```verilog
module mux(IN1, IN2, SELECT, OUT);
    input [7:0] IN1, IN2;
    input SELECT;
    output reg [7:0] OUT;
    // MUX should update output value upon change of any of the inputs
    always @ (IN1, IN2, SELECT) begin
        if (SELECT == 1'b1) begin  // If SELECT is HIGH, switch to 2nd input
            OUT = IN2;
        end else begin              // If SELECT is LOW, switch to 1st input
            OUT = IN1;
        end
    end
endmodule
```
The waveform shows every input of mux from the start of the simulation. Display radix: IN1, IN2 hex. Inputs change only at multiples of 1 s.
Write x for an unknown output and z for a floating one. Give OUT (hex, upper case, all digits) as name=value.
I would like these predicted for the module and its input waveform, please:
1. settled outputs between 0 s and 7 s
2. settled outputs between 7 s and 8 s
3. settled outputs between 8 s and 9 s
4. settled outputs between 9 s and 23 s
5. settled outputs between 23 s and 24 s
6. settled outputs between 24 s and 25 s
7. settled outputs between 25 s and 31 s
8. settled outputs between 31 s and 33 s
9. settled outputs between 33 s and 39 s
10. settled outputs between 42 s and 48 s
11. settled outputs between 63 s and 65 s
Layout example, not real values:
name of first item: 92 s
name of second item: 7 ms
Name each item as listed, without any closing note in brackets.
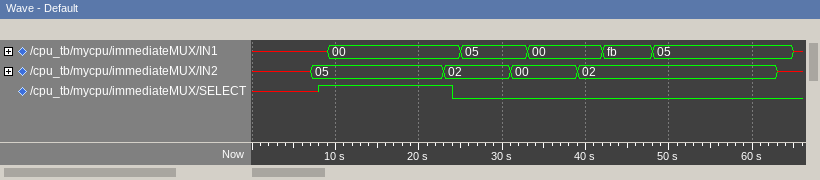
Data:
settled outputs between 0 s and 7 s: OUT=x
settled outputs between 7 s and 8 s: OUT=x
settled outputs between 8 s and 9 s: OUT=05
settled outputs between 9 s and 23 s: OUT=05
settled outputs between 23 s and 24 s: OUT=02
settled outputs between 24 s and 25 s: OUT=00
settled outputs between 25 s and 31 s: OUT=05
settled outputs between 31 s and 33 s: OUT=05
settled outputs between 33 s and 39 s: OUT=00
settled outputs between 42 s and 48 s: OUT=FB
settled outputs between 63 s and 65 s: OUT=05
